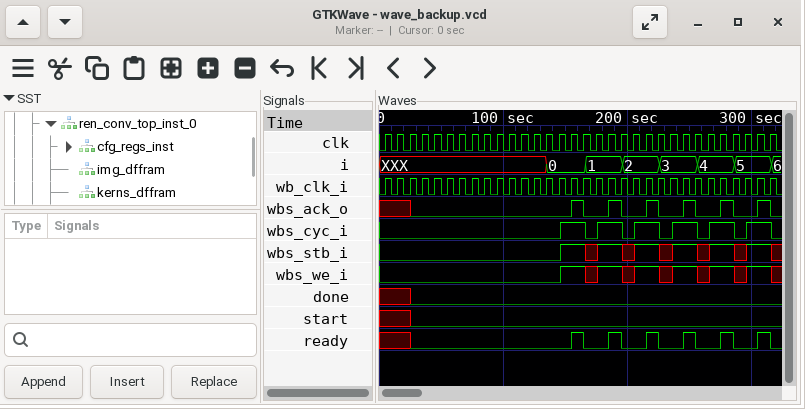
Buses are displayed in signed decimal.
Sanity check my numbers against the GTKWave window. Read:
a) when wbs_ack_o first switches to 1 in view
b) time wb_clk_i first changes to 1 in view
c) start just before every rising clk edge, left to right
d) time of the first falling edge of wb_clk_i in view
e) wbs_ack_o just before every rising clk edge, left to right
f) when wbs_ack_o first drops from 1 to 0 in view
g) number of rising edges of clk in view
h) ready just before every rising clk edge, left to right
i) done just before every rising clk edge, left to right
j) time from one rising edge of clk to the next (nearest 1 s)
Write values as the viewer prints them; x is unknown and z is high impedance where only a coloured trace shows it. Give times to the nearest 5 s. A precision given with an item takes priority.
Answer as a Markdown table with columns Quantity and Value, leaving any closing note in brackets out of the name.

| Quantity | Value |
|---|---|
| when wbs_ack_o first switches to 1 in view | 155 s |
| time wb_clk_i first changes to 1 in view | 5 s |
| start just before every rising clk edge, left to right | x x x 0 0 0 0 0 0 0 0 0 0 0 0 0 0 0 0 0 0 0 0 0 0 0 0 0 0 0 0 0 |
| time of the first falling edge of wb_clk_i in view | 10 s |
| wbs_ack_o just before every rising clk edge, left to right | x x x 0 0 0 0 0 0 0 0 0 0 0 0 0 1 0 0 1 0 0 1 0 0 1 0 0 1 0 0 1 |
| when wbs_ack_o first drops from 1 to 0 in view | 165 s |
| number of rising edges of clk in view | 32 |
| ready just before every rising clk edge, left to right | x x x 0 0 0 0 0 0 0 0 0 0 0 0 0 1 0 0 1 0 0 1 0 0 1 0 0 1 0 0 1 |
| done just before every rising clk edge, left to right | x x x 0 0 0 0 0 0 0 0 0 0 0 0 0 0 0 0 0 0 0 0 0 0 0 0 0 0 0 0 0 |
| time from one rising edge of clk to the next | 10 s |
